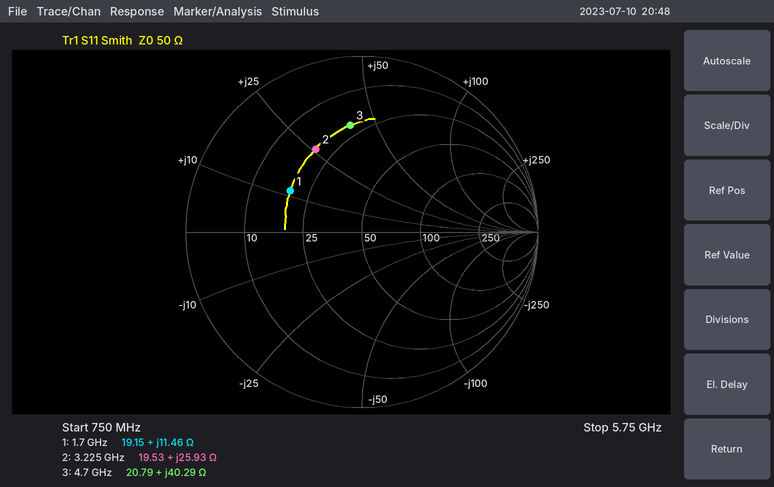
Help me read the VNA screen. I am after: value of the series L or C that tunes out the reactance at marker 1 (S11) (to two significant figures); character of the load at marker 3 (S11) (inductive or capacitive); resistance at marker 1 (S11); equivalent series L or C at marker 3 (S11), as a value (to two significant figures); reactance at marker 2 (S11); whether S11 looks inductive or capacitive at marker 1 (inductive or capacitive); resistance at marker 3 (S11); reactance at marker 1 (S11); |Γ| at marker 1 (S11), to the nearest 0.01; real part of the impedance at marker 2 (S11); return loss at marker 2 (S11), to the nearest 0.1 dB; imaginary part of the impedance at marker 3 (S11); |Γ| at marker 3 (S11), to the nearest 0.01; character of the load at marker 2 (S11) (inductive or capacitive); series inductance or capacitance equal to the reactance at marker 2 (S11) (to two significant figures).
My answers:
8.2 pF
inductive
19.15 Ω
1.4 nH
+25.93 Ω
inductive
20.79 Ω
+11.46 Ω
0.47
19.53 Ω
5.4 dB
+40.29 Ω
0.61
inductive
1.3 nH
